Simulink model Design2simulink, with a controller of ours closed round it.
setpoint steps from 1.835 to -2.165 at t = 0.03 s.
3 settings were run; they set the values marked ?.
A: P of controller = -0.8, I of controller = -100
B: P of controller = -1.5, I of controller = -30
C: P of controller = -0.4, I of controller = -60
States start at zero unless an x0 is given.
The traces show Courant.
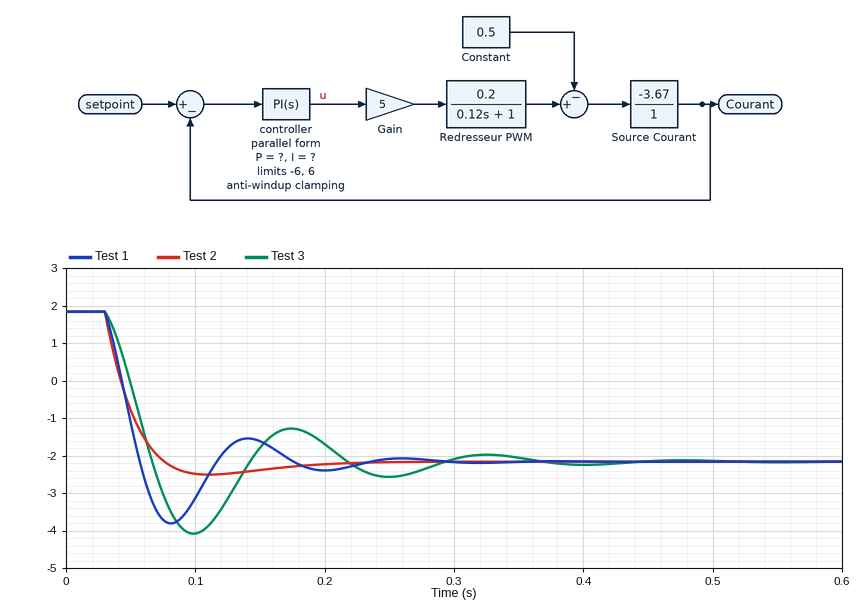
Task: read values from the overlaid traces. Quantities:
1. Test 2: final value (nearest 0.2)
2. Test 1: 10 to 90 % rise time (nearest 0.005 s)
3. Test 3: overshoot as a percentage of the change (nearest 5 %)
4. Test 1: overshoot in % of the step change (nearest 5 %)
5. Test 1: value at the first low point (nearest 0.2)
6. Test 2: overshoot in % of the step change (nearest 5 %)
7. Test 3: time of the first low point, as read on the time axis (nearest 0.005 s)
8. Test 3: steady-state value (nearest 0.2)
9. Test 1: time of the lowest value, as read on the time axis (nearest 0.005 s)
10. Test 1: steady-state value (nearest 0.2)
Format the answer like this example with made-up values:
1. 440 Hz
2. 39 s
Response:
1. -2.2
2. 0.020 s
3. 50 %
4. 40 %
5. -3.8
6. 10 %
7. 0.100 s
8. -2.2
9. 0.080 s
10. -2.2
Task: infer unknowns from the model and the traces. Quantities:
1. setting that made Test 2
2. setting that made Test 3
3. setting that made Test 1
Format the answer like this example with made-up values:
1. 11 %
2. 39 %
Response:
1. B
2. C
3. A
